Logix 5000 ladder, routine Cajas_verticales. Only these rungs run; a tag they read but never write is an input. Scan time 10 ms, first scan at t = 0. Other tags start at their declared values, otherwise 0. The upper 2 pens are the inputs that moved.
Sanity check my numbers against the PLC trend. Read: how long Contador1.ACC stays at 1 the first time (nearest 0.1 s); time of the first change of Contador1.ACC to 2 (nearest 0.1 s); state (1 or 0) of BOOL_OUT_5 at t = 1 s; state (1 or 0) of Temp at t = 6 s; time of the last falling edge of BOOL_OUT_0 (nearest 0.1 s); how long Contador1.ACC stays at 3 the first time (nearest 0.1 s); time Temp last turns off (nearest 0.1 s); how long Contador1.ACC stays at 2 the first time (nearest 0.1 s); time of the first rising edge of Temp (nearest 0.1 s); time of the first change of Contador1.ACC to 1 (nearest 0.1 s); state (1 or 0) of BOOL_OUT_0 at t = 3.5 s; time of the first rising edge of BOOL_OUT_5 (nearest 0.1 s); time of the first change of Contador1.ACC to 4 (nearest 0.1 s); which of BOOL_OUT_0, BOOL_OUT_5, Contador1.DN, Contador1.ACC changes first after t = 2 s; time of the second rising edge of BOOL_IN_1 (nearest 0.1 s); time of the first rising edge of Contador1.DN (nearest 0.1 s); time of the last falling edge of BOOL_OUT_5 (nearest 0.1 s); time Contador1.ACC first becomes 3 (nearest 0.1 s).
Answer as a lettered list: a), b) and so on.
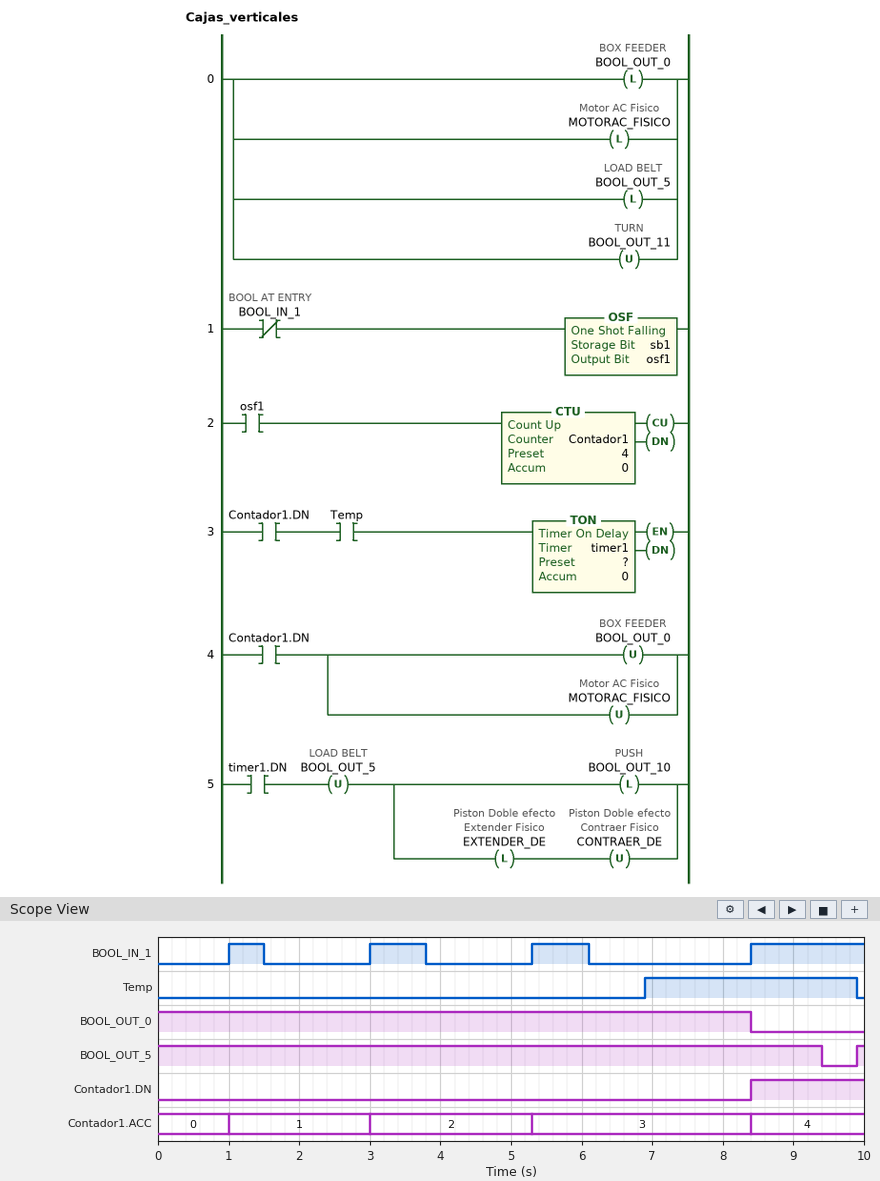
a) 2.0 s
b) 3.0 s
c) 1
d) 0
e) 8.4 s
f) 3.1 s
g) 9.9 s
h) 2.3 s
i) 6.9 s
j) 1.0 s
k) 1
l) 9.9 s
m) 8.4 s
n) Contador1.ACC
o) 3.0 s
p) 8.4 s
q) 9.4 s
r) 5.3 s
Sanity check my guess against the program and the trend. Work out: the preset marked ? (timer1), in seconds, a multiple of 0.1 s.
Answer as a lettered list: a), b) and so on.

a) 1.0 s
